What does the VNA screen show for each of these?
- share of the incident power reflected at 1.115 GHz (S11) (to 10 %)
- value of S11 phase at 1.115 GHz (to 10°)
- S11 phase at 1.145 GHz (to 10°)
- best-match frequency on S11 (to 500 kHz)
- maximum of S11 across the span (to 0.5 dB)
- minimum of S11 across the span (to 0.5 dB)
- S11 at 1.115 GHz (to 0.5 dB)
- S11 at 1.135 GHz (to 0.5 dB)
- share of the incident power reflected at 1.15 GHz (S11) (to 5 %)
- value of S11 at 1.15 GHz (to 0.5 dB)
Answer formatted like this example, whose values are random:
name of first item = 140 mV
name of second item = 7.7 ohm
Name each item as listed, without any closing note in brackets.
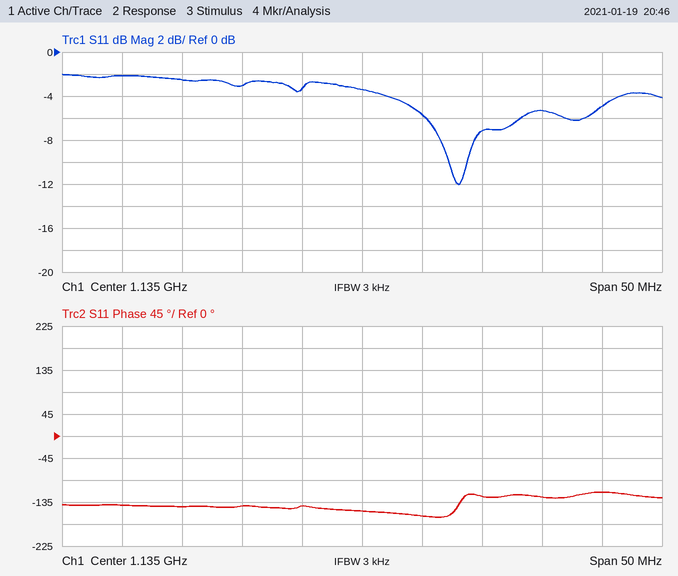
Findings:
share of the incident power reflected at 1.115 GHz (S11) = 60 %
value of S11 phase at 1.115 GHz = -140°
S11 phase at 1.145 GHz = -120°
best-match frequency on S11 = 1.1430 GHz
maximum of S11 across the span = -2.0 dB
minimum of S11 across the span = -12.0 dB
S11 at 1.115 GHz = -2.0 dB
S11 at 1.135 GHz = -3.5 dB
share of the incident power reflected at 1.15 GHz (S11) = 30 %
value of S11 at 1.15 GHz = -5.5 dB
